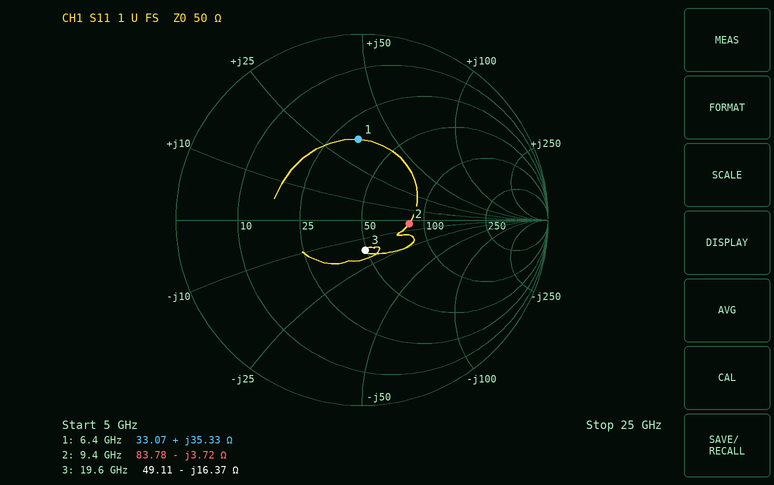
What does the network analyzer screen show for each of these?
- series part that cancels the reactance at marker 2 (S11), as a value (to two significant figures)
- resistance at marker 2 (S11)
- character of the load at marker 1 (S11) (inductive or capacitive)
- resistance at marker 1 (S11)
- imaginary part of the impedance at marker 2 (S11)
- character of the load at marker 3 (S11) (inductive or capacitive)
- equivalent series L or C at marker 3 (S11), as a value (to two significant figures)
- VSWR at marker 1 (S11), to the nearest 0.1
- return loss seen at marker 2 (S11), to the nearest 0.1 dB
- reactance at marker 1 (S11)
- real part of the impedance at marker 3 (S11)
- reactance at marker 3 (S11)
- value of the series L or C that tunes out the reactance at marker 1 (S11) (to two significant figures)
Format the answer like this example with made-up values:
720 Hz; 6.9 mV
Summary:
63 pH; 83.78 Ω; inductive; 33.07 Ω; -3.72 Ω; capacitive; 500 fF; 2.5; 11.9 dB; +35.33 Ω; 49.11 Ω; -16.37 Ω; 700 fF
